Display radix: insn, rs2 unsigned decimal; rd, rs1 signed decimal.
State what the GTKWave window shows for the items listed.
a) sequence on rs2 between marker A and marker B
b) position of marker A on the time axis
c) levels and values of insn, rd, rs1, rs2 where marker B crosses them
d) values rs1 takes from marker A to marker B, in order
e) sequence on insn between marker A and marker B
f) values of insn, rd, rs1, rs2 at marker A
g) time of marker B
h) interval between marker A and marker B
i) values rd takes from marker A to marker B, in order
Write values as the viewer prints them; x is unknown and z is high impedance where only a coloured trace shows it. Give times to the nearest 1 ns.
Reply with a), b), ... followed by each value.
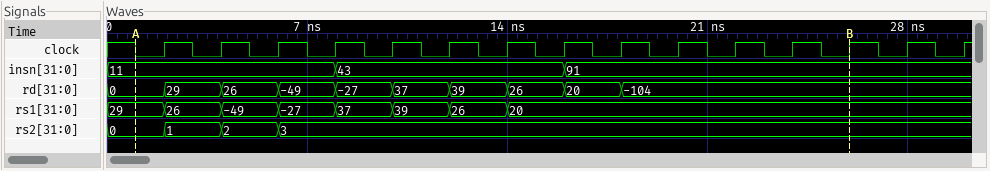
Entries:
a) 0, 1, 2, 3
b) 1 ns
c) insn=91, rd=-104, rs1=20, rs2=3
d) 29, 26, -49, -27, 37, 39, 26, 20
e) 11, 43, 91
f) insn=11, rd=0, rs1=29, rs2=0
g) 26 ns
h) 25 ns
i) 0, 29, 26, -49, -27, 37, 39, 26, 20, -104
